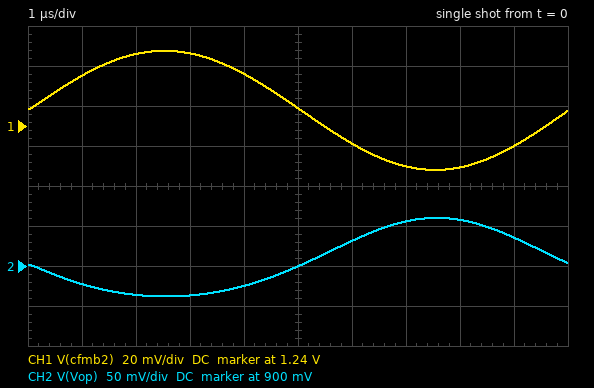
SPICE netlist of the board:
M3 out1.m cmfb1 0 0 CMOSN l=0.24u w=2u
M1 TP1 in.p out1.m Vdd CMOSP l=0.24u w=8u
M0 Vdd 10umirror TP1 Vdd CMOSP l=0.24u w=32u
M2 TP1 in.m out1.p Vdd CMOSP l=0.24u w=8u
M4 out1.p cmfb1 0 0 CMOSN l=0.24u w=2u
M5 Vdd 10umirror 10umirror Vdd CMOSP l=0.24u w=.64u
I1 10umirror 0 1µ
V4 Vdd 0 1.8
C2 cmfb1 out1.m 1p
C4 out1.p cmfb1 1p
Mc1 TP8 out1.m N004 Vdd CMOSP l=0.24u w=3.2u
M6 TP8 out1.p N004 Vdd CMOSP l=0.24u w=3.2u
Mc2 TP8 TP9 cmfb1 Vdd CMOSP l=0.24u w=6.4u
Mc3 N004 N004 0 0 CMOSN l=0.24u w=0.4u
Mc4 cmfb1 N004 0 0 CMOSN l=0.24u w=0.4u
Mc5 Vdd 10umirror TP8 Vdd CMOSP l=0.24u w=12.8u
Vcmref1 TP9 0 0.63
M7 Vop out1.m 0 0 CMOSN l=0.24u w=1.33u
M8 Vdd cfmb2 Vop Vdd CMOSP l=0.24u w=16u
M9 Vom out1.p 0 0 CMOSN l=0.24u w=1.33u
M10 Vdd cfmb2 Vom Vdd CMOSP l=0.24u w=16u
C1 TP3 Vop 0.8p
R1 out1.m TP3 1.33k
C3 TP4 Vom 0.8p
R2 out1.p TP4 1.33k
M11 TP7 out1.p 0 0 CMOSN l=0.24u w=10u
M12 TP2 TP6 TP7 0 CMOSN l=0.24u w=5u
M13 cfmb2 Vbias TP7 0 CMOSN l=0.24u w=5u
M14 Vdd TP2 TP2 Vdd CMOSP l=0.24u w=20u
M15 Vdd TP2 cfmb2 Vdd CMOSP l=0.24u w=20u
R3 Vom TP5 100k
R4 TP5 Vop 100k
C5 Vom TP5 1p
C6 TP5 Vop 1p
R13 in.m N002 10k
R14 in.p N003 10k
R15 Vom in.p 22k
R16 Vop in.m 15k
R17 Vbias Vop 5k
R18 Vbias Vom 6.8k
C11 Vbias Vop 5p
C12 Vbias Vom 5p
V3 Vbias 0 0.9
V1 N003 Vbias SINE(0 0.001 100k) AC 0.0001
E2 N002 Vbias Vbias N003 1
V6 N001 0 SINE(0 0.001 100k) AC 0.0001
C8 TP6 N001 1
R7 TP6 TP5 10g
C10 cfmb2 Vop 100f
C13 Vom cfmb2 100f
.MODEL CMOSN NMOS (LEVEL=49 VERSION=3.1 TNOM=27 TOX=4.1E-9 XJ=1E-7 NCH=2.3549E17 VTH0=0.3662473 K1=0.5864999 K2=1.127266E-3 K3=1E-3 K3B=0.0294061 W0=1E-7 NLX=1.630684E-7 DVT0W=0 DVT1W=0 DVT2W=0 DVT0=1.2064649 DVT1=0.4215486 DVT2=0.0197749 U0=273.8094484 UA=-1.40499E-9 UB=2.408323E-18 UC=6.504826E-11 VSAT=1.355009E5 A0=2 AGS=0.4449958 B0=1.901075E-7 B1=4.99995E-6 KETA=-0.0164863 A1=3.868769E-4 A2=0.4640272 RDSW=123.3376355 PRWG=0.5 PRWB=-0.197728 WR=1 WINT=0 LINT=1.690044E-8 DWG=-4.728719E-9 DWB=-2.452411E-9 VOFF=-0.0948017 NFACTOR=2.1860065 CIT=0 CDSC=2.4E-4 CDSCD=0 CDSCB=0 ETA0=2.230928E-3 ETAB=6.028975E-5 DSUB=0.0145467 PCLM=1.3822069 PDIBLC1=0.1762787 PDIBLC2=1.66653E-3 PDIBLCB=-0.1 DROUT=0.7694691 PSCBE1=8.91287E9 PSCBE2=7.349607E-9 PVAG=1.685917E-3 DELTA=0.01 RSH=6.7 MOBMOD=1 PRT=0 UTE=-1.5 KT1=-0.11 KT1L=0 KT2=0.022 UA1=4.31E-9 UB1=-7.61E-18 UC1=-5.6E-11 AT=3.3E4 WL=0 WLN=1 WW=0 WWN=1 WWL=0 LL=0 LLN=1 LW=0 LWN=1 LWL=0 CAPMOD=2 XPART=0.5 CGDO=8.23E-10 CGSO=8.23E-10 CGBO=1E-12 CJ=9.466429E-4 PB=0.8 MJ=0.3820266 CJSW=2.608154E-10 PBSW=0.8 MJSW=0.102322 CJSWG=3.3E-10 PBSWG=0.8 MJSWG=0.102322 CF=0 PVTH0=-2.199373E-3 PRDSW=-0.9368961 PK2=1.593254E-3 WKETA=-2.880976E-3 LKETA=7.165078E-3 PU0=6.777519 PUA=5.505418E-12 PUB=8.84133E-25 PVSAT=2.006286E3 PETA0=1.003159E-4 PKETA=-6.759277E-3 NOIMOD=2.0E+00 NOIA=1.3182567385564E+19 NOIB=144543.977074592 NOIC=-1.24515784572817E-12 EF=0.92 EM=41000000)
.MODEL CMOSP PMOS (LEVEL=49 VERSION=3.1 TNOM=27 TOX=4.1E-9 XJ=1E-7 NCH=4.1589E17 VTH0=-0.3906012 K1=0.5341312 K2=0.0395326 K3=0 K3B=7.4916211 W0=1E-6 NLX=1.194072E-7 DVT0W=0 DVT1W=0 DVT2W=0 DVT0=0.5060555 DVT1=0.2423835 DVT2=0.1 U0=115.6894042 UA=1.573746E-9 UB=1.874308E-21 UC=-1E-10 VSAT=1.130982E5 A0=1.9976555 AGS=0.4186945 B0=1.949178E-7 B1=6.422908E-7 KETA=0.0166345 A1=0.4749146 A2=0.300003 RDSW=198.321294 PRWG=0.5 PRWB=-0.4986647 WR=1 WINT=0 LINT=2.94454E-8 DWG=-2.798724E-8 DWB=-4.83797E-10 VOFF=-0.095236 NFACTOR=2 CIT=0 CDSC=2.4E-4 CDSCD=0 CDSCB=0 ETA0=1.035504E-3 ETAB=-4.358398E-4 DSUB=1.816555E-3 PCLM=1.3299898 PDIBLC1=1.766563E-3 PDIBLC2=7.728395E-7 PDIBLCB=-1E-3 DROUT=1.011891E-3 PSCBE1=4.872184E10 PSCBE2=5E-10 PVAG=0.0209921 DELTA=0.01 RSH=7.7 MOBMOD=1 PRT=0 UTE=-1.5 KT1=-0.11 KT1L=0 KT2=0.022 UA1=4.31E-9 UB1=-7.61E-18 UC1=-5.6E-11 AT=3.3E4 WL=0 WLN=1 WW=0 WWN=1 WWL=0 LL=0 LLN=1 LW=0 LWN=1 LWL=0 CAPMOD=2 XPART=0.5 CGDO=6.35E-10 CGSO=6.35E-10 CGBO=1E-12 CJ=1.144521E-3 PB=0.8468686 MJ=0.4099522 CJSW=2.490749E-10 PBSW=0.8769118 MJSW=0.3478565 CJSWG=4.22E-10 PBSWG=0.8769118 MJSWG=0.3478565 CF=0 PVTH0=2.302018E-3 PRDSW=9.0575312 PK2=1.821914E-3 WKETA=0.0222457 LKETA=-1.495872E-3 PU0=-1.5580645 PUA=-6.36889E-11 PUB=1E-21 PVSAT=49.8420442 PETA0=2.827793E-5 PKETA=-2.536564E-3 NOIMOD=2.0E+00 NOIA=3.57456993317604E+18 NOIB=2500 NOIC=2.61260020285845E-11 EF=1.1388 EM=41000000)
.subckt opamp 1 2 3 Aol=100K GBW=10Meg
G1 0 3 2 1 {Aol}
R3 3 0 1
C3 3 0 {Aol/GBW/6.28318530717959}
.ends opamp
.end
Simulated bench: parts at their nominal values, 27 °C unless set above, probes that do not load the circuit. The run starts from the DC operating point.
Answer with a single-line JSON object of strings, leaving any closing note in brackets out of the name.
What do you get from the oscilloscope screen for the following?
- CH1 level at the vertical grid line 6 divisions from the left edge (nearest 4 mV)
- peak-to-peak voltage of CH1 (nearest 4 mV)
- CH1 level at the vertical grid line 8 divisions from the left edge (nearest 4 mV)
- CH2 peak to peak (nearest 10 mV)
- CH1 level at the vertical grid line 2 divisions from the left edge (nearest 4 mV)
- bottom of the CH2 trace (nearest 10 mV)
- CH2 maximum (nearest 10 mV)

{"CH1 level at the vertical grid line 6 divisions from the left edge": "1.232 V", "peak-to-peak voltage of CH1": "60 mV", "CH1 level at the vertical grid line 8 divisions from the left edge": "1.220 V", "CH2 peak to peak": "100 mV", "CH1 level at the vertical grid line 2 divisions from the left edge": "1.276 V", "bottom of the CH2 trace": "860 mV", "CH2 maximum": "960 mV"}
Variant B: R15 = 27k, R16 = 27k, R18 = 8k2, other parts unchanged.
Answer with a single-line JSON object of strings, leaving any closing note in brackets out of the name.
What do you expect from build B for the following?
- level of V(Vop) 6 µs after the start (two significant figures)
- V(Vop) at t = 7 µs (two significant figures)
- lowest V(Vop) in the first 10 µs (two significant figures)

{"level of V(Vop) 6 µs after the start": "950 mV", "V(Vop) at t = 7 µs": "1.0 V", "lowest V(Vop) in the first 10 µs": "840 mV"}
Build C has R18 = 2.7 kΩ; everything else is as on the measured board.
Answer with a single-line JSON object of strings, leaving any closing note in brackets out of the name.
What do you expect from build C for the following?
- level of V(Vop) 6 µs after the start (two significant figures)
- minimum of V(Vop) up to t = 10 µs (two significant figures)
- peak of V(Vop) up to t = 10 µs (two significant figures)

{"level of V(Vop) 6 µs after the start": "910 mV", "minimum of V(Vop) up to t = 10 µs": "880 mV", "peak of V(Vop) up to t = 10 µs": "920 mV"}
